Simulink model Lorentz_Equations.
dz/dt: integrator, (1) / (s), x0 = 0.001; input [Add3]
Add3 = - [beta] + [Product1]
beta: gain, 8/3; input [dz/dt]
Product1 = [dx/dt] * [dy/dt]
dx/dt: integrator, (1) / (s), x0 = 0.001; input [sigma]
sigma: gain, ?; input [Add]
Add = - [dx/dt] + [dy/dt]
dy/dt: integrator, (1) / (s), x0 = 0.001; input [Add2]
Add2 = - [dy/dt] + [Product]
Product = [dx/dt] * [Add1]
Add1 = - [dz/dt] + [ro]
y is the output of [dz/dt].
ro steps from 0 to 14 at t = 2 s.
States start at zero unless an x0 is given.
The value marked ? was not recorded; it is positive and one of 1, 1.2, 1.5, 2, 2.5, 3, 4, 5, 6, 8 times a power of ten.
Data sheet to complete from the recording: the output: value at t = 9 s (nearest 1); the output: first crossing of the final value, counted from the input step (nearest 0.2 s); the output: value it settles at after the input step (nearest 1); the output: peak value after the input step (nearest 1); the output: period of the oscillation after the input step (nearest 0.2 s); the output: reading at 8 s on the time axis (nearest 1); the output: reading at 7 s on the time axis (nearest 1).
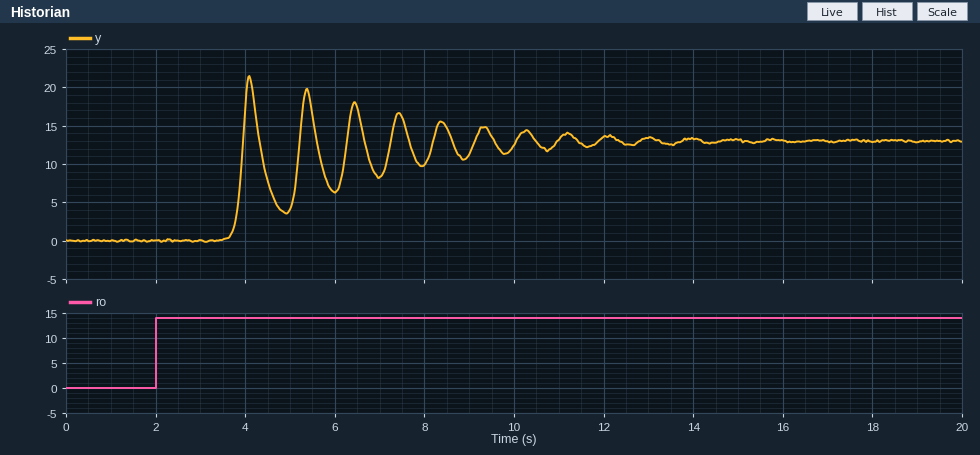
11
2.0 s
13
21
1.2 s
10
8
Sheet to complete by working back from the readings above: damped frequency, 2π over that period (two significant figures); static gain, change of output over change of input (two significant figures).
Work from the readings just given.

5.2 rad/s
0.93
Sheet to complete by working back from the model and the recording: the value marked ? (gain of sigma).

6
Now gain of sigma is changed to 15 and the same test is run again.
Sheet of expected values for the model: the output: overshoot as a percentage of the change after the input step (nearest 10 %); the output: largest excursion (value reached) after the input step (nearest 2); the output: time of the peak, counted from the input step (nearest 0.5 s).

70 %
22
1.5 s
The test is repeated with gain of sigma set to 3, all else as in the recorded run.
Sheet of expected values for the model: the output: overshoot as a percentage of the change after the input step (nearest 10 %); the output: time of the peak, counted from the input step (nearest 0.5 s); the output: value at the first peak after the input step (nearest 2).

60 %
2.5 s
20
